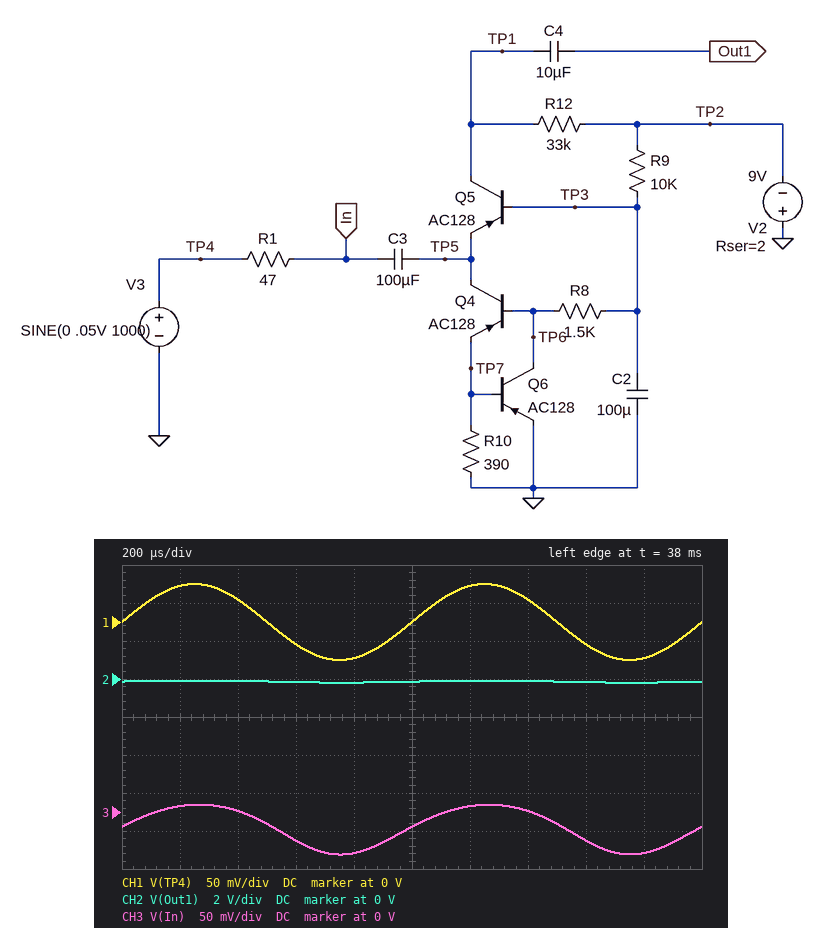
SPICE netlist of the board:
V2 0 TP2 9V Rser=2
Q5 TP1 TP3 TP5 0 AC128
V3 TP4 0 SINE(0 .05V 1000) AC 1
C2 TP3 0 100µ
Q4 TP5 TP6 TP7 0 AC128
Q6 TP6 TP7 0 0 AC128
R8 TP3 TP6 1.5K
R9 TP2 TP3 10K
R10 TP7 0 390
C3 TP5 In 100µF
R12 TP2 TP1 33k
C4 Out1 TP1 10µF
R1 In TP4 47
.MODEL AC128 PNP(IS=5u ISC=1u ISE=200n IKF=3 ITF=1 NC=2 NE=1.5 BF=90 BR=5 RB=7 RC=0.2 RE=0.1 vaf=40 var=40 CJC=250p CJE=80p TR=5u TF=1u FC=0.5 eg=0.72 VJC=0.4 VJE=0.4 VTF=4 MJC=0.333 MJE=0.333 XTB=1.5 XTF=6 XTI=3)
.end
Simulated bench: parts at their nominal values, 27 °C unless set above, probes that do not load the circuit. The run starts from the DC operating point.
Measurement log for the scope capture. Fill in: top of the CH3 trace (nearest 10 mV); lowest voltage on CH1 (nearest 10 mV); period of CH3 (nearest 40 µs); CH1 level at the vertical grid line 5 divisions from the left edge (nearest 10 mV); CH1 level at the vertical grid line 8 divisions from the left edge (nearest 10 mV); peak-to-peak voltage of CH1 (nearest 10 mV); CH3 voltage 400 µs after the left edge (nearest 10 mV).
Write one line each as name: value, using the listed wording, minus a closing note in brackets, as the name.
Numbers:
top of the CH3 trace: 10 mV
lowest voltage on CH1: -50 mV
period of CH3: 1.00 ms
CH1 level at the vertical grid line 5 divisions from the left edge: 0 V
CH1 level at the vertical grid line 8 divisions from the left edge: -30 mV
peak-to-peak voltage of CH1: 100 mV
CH3 voltage 400 µs after the left edge: 0 V
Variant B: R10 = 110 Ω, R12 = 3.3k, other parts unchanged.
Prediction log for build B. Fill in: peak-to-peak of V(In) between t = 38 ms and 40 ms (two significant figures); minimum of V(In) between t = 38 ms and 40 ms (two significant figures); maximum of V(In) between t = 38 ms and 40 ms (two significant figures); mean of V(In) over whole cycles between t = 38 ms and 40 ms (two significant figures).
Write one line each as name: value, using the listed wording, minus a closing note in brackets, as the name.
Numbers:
peak-to-peak of V(In) between t = 38 ms and 40 ms: 33 mV
minimum of V(In) between t = 38 ms and 40 ms: -51 mV
maximum of V(In) between t = 38 ms and 40 ms: -18 mV
mean of V(In) over whole cycles between t = 38 ms and 40 ms: -33 mV
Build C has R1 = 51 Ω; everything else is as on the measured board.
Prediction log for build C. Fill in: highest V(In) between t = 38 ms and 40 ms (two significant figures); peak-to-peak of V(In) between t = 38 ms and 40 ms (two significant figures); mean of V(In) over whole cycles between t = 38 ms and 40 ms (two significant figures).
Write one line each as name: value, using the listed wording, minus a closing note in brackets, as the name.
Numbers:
highest V(In) between t = 38 ms and 40 ms: 7.0 mV
peak-to-peak of V(In) between t = 38 ms and 40 ms: 64 mV
mean of V(In) over whole cycles between t = 38 ms and 40 ms: -22 mV
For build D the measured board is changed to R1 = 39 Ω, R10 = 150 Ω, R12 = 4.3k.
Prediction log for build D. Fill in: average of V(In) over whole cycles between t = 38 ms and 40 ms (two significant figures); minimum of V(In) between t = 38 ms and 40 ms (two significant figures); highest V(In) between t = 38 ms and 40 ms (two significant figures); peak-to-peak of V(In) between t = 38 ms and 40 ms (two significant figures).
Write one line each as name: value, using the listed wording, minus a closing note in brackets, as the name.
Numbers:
average of V(In) over whole cycles between t = 38 ms and 40 ms: -28 mV
minimum of V(In) between t = 38 ms and 40 ms: -50 mV
highest V(In) between t = 38 ms and 40 ms: -9.3 mV
peak-to-peak of V(In) between t = 38 ms and 40 ms: 41 mV
